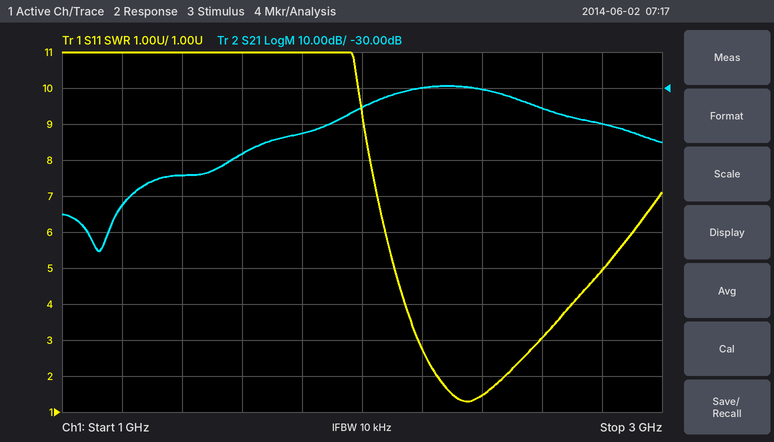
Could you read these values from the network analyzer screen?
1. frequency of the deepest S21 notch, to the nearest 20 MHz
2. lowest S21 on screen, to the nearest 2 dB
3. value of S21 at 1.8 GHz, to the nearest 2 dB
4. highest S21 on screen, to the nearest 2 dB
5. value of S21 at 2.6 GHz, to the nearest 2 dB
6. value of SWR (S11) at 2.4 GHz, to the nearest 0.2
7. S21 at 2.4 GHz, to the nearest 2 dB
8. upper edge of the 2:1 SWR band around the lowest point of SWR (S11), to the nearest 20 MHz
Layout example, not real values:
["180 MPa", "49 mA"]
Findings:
["1.12 GHz", "-76 dB", "-42 dB", "-30 dB", "-36 dB", "1.4", "-30 dB", "2.48 GHz"]
